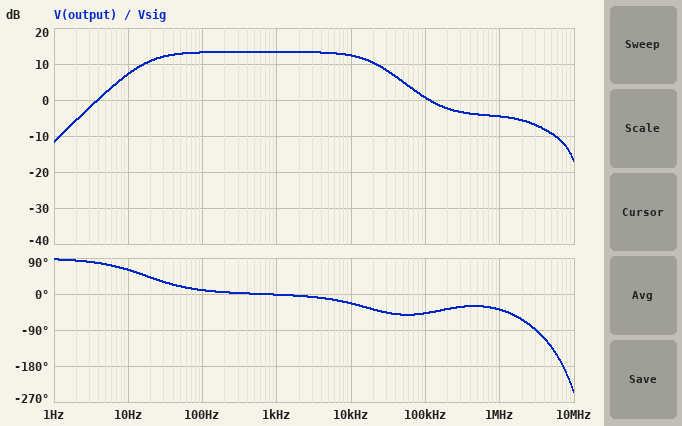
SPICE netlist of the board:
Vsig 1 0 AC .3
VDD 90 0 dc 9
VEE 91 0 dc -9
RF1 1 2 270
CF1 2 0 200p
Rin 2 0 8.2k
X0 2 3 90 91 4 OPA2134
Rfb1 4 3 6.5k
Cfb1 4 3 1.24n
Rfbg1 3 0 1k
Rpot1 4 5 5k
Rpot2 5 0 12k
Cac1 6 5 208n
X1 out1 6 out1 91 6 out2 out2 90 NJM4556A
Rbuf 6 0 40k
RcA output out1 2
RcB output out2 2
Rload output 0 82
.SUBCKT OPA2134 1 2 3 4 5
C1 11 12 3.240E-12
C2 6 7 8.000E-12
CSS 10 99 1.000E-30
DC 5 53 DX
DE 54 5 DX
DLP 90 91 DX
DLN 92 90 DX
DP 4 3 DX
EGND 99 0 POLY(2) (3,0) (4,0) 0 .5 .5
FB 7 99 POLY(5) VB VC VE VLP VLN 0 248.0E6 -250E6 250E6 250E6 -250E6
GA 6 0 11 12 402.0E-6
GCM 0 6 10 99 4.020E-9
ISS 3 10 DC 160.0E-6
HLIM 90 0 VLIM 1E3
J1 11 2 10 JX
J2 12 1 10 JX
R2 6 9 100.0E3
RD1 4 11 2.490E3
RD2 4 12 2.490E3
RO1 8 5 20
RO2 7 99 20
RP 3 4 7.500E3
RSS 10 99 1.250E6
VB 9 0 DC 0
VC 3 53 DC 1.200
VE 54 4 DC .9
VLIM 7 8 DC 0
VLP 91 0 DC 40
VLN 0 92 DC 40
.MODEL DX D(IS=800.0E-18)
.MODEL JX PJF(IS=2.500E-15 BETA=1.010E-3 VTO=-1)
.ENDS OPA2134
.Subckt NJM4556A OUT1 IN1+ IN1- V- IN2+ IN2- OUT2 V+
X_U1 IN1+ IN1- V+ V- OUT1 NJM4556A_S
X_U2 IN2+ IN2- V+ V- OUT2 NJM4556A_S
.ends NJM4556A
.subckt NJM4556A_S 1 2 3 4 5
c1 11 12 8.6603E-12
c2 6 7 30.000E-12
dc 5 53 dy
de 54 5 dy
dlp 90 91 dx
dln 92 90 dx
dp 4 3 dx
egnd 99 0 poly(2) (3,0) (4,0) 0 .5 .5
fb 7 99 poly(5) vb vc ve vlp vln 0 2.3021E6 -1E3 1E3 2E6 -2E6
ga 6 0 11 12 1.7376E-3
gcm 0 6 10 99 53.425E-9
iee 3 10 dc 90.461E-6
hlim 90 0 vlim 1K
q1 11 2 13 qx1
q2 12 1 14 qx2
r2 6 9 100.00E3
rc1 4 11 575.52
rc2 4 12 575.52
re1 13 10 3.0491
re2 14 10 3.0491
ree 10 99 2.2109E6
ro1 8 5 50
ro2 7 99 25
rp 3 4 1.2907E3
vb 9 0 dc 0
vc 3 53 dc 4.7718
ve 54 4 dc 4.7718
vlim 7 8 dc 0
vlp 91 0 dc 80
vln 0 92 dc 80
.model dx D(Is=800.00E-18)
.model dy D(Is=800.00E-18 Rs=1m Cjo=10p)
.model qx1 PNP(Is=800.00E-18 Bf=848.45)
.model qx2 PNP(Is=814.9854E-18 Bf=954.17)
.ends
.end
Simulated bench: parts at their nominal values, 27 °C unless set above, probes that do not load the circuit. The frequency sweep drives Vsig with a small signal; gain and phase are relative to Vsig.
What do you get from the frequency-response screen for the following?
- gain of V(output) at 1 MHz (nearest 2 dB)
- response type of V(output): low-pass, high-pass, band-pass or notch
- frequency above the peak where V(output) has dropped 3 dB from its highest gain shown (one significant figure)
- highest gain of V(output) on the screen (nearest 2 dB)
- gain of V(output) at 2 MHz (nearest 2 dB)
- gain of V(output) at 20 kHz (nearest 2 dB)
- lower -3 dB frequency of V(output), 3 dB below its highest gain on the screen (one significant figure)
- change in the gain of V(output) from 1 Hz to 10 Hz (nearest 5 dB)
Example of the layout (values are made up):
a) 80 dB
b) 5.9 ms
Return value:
a) -4 dB
b) band-pass
c) 20 kHz
d) 14 dB
e) -6 dB
f) 10 dB
g) 20 Hz
h) 20 dB
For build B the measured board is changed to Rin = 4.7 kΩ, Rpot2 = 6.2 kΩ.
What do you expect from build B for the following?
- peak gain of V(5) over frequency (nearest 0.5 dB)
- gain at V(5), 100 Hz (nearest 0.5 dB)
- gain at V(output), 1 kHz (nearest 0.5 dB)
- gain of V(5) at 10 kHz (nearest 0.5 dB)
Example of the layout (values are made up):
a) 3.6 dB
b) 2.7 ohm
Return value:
a) 12.0 dB
b) 11.5 dB
c) 11.0 dB
d) 10.5 dB
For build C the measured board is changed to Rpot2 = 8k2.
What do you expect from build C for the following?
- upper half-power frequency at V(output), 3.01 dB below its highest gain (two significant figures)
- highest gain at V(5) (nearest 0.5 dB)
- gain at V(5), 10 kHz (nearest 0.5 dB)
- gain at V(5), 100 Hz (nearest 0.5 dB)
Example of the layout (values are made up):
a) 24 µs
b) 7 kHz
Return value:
a) 20 kHz
b) 13.0 dB
c) 11.5 dB
d) 12.5 dB
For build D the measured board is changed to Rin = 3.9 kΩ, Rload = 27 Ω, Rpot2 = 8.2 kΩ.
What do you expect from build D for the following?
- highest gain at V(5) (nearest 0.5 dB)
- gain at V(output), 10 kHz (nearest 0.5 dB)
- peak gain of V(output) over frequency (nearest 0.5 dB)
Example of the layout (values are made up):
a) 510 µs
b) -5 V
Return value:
a) 13.0 dB
b) 11.0 dB
c) 12.0 dB
